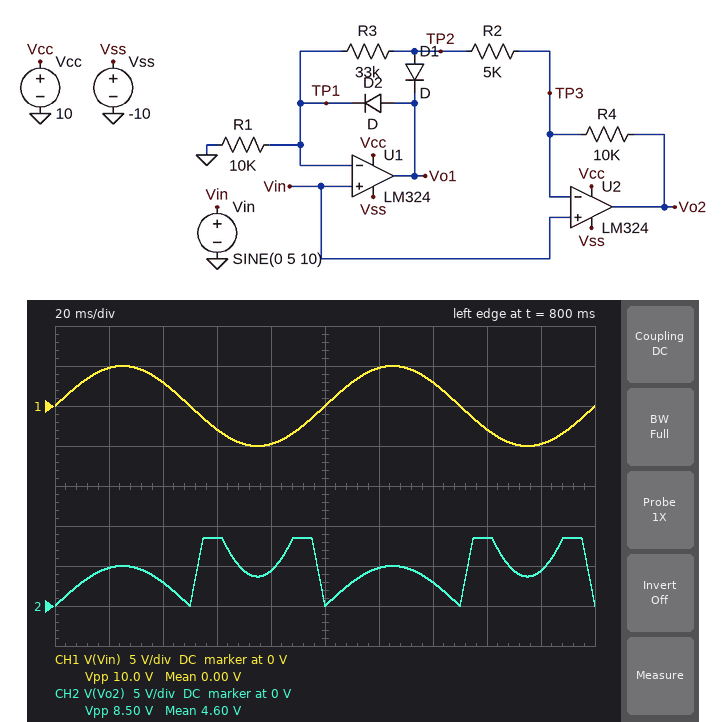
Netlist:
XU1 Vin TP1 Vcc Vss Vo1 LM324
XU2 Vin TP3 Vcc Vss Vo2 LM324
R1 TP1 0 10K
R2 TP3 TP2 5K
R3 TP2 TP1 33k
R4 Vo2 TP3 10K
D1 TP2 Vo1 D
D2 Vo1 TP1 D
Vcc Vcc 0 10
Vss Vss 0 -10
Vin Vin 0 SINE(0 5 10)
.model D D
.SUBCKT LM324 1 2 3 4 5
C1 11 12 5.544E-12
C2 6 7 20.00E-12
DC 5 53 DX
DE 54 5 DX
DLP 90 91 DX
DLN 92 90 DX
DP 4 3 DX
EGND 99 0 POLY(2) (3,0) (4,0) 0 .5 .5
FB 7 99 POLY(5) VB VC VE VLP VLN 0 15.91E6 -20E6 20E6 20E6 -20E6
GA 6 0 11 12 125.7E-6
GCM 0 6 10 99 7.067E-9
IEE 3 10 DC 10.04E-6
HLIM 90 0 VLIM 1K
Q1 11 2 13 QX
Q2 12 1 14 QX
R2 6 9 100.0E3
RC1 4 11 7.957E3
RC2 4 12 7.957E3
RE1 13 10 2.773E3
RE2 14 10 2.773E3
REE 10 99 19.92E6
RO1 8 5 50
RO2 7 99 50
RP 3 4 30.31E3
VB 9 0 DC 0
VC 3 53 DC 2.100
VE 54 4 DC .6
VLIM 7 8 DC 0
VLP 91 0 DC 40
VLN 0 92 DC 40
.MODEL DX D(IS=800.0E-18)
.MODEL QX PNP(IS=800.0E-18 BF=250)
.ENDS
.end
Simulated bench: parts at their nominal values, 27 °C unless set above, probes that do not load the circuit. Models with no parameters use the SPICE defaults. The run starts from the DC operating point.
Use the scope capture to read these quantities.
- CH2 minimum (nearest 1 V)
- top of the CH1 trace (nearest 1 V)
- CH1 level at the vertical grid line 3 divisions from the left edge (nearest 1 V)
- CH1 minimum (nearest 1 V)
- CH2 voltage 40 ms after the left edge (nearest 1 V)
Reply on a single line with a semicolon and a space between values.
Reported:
0 V; 5 V; -3 V; -5 V; 3 V
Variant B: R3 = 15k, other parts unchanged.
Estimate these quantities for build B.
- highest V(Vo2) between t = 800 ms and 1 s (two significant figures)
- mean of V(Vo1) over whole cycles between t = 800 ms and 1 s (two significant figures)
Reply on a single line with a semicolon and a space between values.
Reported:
7.4 V; -1.9 V
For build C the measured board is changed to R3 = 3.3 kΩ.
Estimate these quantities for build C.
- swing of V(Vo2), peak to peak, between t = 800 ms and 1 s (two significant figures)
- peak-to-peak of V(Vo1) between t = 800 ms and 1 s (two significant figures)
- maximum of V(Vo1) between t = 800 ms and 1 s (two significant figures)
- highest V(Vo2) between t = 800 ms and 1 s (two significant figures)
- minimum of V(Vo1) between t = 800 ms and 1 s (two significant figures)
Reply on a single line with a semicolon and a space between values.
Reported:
6.7 V; 13 V; 5.6 V; 5.0 V; -7.3 V
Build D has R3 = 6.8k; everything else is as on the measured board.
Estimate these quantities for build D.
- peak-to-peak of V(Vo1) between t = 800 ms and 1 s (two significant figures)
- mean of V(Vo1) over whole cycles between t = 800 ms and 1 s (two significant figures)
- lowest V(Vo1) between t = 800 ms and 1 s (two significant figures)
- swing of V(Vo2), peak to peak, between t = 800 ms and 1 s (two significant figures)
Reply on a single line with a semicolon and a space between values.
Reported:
15 V; -1.1 V; -9.1 V; 5.0 V
